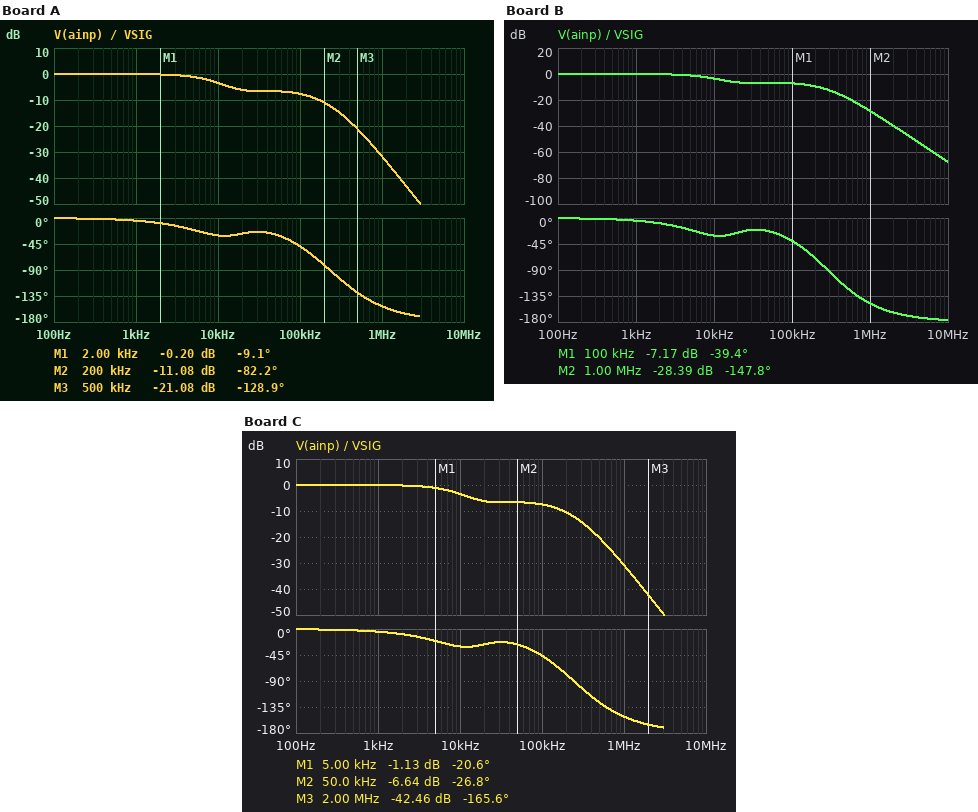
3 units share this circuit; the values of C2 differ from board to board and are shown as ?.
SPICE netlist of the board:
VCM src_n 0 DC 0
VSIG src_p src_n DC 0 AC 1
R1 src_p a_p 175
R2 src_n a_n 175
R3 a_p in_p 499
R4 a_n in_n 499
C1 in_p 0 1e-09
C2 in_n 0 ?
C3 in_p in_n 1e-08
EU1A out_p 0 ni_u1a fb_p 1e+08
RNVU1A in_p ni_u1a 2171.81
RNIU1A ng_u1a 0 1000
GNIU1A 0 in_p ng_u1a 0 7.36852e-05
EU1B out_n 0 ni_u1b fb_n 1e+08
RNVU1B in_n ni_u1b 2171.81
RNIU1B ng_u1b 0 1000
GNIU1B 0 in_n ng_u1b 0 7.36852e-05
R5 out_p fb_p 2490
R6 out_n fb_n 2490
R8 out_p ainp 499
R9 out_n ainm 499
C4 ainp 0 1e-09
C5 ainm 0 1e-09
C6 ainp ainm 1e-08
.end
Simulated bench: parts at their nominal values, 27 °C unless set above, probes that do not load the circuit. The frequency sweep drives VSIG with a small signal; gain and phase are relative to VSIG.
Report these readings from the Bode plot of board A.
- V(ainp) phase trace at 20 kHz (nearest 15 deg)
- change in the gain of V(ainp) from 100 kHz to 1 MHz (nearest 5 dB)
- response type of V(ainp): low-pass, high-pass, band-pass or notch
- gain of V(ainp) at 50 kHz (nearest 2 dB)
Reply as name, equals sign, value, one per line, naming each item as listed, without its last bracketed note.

V(ainp) phase trace at 20 kHz = -30 deg
change in the gain of V(ainp) from 100 kHz to 1 MHz = -25 dB
response type of V(ainp): low-pass, high-pass, band-pass or notch = low-pass
gain of V(ainp) at 50 kHz = -6 dB
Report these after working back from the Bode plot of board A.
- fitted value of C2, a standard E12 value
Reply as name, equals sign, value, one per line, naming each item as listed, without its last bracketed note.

fitted value of C2, a standard E12 value = 1.8 nF
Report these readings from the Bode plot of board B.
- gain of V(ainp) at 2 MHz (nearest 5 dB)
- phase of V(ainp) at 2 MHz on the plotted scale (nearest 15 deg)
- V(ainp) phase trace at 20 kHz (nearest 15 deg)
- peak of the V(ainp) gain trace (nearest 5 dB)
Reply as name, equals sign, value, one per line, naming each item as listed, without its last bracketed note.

gain of V(ainp) at 2 MHz = -40 dB
phase of V(ainp) at 2 MHz on the plotted scale = -165 deg
V(ainp) phase trace at 20 kHz = -30 deg
peak of the V(ainp) gain trace = 0 dB
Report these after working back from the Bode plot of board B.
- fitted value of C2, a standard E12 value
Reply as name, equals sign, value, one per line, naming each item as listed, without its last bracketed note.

fitted value of C2, a standard E12 value = 820 pF
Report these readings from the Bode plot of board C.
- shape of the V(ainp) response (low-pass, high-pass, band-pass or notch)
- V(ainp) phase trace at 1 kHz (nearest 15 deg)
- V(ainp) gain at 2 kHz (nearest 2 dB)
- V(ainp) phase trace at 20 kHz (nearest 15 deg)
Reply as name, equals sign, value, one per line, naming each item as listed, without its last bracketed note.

shape of the V(ainp) response = low-pass
V(ainp) phase trace at 1 kHz = 0 deg
V(ainp) gain at 2 kHz = 0 dB
V(ainp) phase trace at 20 kHz = -30 deg
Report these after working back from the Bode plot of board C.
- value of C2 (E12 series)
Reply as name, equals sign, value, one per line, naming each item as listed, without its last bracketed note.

value of C2 = 1.5 nF
